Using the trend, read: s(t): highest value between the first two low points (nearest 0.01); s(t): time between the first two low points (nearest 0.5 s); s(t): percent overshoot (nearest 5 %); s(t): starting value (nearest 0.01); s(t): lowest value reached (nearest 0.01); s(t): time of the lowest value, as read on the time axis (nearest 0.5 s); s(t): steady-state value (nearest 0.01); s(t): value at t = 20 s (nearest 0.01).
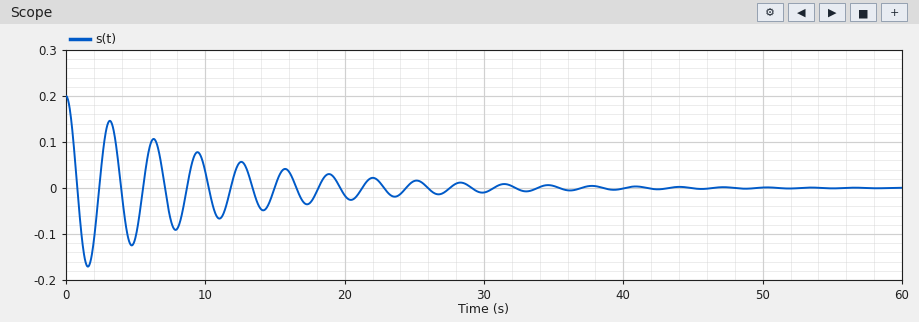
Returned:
0.15
3.0 s
85 %
0.20
-0.17
1.5 s
0.00
-0.02
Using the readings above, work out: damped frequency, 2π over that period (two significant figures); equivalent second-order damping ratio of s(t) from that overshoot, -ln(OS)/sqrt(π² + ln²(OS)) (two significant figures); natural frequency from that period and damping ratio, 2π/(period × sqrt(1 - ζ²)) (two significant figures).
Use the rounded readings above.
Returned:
2.1 rad/s
0.052
2.1 rad/s
